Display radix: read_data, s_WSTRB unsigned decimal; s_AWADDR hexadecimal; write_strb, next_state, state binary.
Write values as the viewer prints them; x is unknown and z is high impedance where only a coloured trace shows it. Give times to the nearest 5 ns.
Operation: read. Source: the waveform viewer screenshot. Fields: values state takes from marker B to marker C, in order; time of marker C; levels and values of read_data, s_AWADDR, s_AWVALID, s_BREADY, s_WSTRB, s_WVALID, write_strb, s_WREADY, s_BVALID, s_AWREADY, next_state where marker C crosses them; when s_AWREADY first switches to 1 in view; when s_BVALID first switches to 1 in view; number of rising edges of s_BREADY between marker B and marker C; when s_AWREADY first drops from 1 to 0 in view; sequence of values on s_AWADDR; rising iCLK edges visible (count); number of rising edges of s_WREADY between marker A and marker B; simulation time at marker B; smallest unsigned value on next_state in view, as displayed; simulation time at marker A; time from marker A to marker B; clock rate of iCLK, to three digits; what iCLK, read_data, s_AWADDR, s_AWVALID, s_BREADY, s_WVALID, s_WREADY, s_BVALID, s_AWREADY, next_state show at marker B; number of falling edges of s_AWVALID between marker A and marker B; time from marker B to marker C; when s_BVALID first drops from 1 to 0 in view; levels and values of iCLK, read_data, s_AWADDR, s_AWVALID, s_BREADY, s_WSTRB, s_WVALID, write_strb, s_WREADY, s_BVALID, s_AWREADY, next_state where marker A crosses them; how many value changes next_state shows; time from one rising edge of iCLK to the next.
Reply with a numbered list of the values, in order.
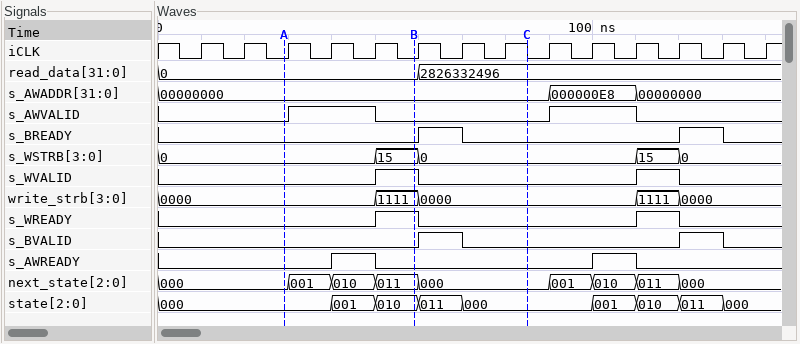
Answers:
1. 010, 011, 000
2. 85 ns
3. read_data=2826332496, s_AWADDR=00000000, s_AWVALID=0, s_BREADY=0, s_WSTRB=0, s_WVALID=0, write_strb=0000, s_WREADY=0, s_BVALID=0, s_AWREADY=0, next_state=000
4. 40 ns
5. 60 ns
6. 1
7. 50 ns
8. 00000000, 000000E8, 00000000
9. 14
10. 1
11. 60 ns
12. 000
13. 30 ns
14. 30 ns
15. 100 MHz
16. iCLK=0, read_data=0, s_AWADDR=00000000, s_AWVALID=0, s_BREADY=0, s_WVALID=1, s_WREADY=1, s_BVALID=0, s_AWREADY=0, next_state=011
17. 1
18. 25 ns
19. 70 ns
20. iCLK=0, read_data=0, s_AWADDR=00000000, s_AWVALID=0, s_BREADY=0, s_WSTRB=0, s_WVALID=0, write_strb=0000, s_WREADY=0, s_BVALID=0, s_AWREADY=0, next_state=000
21. 8
22. 10 ns
